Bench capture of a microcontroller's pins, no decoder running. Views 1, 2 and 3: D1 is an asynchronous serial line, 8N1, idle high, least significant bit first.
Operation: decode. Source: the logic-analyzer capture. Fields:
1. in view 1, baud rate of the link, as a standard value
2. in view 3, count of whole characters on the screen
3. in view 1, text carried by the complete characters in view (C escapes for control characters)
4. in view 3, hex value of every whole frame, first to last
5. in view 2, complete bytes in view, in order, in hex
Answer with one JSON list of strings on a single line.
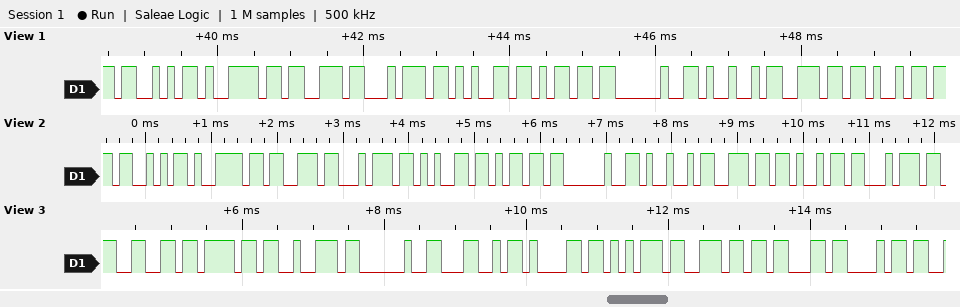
["9600 baud", "10", "\"System Ini\"", "66 6F 72 20 4C 61 75 6E 63 68", "53 79 73 74 65 6D 20 49 6E 69 74"]
